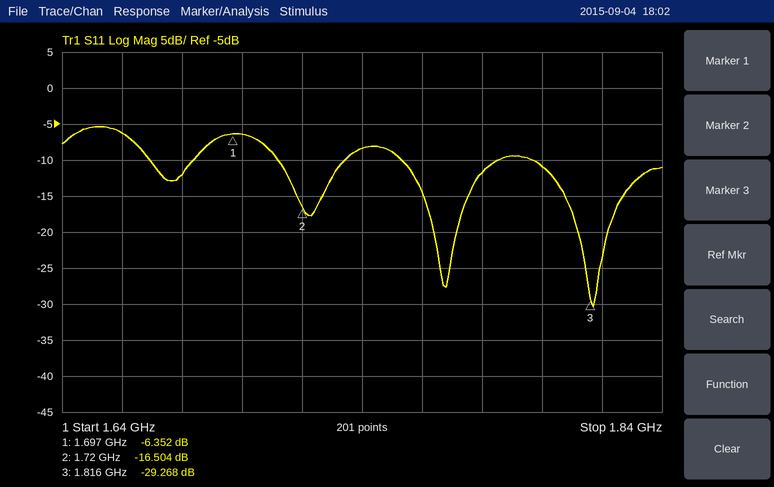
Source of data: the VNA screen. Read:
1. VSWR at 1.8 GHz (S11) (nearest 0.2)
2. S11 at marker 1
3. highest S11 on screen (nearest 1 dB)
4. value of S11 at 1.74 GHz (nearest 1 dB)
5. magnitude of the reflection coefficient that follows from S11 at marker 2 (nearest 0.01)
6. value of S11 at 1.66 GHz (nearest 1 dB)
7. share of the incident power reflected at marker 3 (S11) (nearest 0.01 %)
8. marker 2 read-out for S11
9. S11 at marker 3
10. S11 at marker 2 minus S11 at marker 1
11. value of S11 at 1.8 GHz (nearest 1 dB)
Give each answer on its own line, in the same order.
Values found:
1.8
-6.352 dB
-5 dB
-8 dB
0.15
-6 dB
0.12 %
-16.504 dB
-29.268 dB
-10.152 dB
-11 dB
